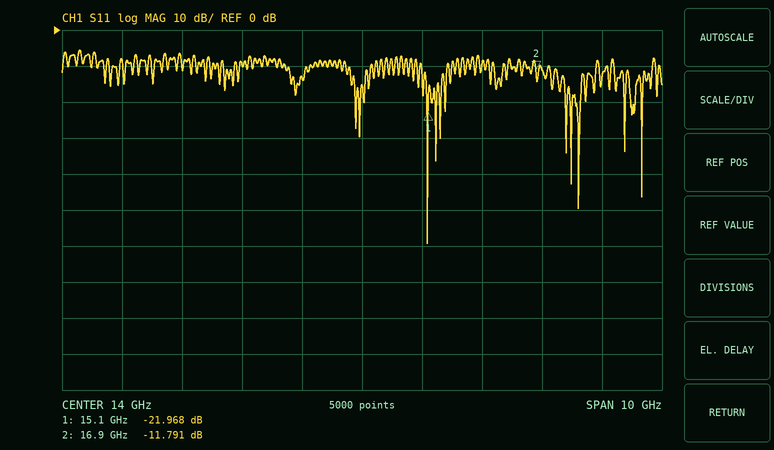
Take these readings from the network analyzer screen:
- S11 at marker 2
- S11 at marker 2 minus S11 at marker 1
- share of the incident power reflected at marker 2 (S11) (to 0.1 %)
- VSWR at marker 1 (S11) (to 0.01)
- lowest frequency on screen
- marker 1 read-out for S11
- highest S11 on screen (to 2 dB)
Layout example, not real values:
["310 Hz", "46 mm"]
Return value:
["-11.791 dB", "10.177 dB", "6.6 %", "1.17", "9 GHz", "-21.968 dB", "-6 dB"]
